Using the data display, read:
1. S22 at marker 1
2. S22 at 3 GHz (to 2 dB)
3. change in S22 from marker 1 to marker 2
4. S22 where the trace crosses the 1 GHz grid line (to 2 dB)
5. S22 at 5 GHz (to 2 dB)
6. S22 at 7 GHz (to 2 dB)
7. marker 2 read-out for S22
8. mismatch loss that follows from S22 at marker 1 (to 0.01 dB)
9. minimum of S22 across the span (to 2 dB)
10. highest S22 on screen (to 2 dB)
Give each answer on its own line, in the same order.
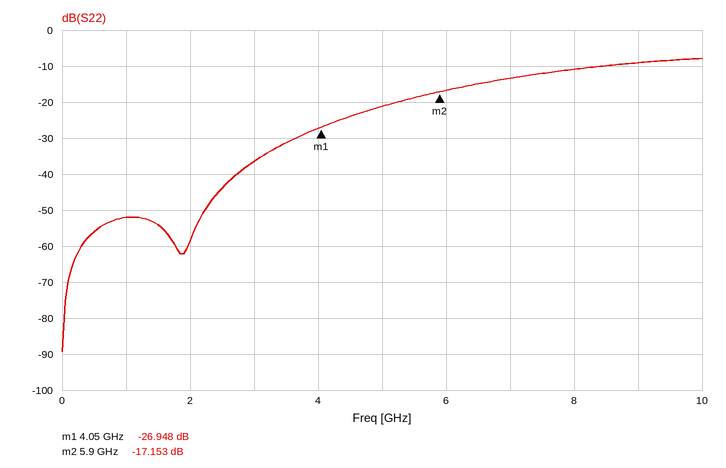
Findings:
-26.948 dB
-36 dB
9.795 dB
-52 dB
-22 dB
-14 dB
-17.153 dB
0.01 dB
-90 dB
-8 dB
